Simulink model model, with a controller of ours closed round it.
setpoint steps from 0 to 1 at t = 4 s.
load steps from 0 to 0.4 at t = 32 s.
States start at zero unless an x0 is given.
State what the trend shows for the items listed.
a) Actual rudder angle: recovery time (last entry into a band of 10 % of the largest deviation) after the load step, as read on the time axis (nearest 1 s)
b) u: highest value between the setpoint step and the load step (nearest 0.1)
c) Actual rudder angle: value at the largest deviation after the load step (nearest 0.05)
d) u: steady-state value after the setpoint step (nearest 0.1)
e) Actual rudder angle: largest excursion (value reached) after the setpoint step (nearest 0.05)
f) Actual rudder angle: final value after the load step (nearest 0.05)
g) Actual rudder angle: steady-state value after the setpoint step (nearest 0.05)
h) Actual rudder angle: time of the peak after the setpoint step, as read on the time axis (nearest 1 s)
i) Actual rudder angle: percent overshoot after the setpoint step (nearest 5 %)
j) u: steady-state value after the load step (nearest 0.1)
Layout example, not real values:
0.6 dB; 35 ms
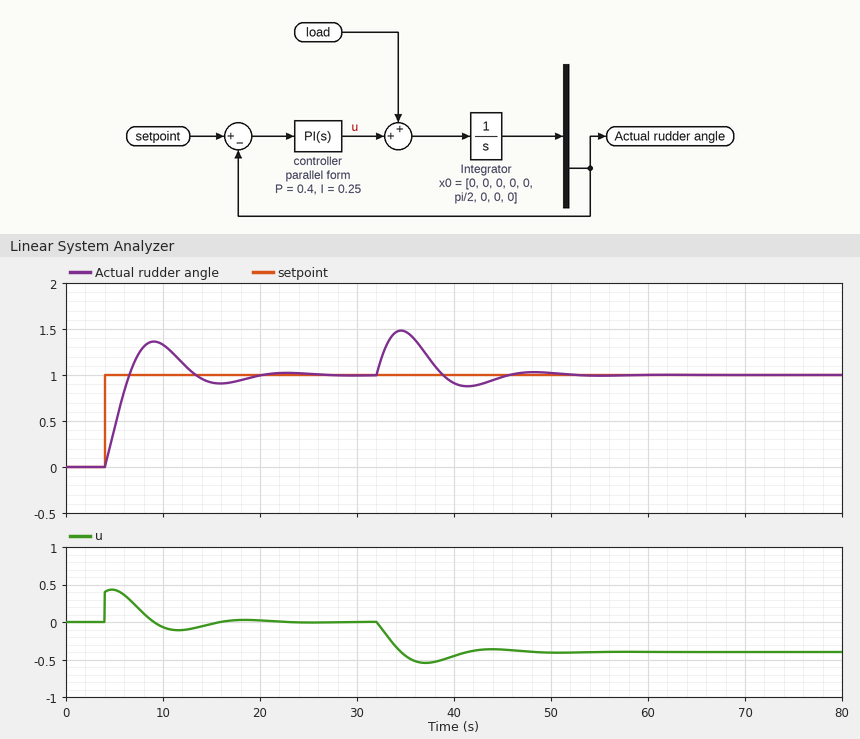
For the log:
44 s; 0.4; 1.50; 0.0; 1.35; 1.00; 1.00; 9 s; 35 %; -0.4
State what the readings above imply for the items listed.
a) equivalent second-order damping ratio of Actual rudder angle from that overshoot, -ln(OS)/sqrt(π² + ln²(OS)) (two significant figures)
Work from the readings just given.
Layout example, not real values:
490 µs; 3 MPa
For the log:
0.32
